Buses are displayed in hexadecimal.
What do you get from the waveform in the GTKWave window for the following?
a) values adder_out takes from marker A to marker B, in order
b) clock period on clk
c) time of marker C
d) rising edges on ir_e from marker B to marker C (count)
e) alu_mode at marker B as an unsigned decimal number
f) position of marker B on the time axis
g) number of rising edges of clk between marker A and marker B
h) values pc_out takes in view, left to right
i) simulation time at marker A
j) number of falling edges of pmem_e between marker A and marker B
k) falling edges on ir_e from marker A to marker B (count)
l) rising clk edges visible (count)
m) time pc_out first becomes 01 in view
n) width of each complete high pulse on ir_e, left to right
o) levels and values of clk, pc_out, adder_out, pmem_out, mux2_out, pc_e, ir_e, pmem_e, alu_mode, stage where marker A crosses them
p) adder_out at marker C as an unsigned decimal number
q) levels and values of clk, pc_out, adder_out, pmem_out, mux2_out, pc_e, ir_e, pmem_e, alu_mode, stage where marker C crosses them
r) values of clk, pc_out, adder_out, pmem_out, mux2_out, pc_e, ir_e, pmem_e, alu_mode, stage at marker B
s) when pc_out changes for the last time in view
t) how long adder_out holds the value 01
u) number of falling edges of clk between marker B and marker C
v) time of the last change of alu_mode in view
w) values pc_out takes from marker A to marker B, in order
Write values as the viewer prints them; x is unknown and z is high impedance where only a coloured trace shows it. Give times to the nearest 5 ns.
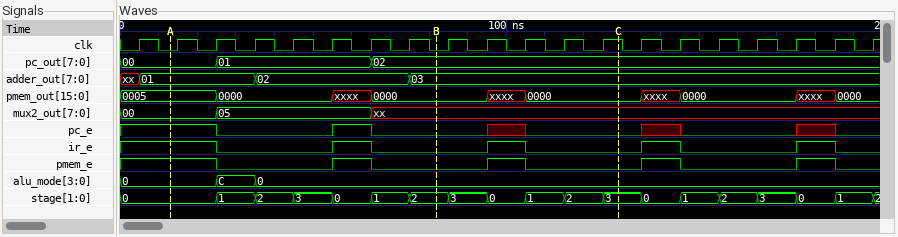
01, 02, 03
10 ns
130 ns
1
0
80 ns
7
00, 01, 02
15 ns
2
2
20
25 ns
10 ns, 10 ns, 10 ns, 10 ns
clk=0, pc_out=00, adder_out=01, pmem_out=0005, mux2_out=00, pc_e=1, ir_e=1, pmem_e=1, alu_mode=0, stage=0
3
clk=1, pc_out=02, adder_out=03, pmem_out=0000, mux2_out=xx, pc_e=0, ir_e=0, pmem_e=0, alu_mode=0, stage=3
clk=0, pc_out=02, adder_out=03, pmem_out=0000, mux2_out=xx, pc_e=0, ir_e=0, pmem_e=0, alu_mode=0, stage=2
65 ns
30 ns
4
35 ns
00, 01, 02
